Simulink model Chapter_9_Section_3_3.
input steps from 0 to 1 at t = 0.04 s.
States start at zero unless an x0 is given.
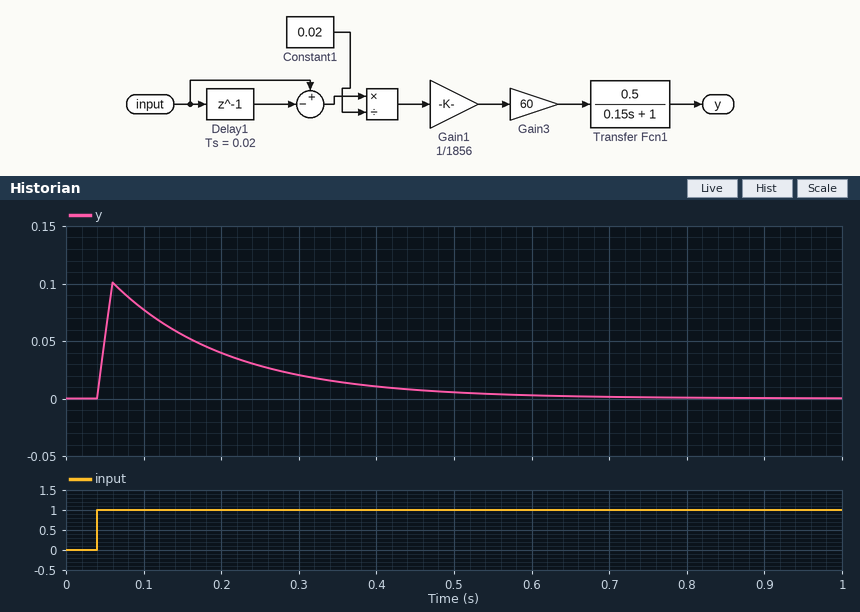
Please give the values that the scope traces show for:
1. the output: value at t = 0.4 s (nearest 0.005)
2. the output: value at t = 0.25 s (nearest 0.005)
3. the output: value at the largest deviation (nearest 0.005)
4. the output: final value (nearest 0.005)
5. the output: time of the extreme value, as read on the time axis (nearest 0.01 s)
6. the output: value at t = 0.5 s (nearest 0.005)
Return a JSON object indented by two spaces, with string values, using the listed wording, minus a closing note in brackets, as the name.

{
  "the output: value at t = 0.4 s": "0.010",
  "the output: value at t = 0.25 s": "0.030",
  "the output: value at the largest deviation": "0.100",
  "the output: final value": "0.000",
  "the output: time of the extreme value, as read on the time axis": "0.06 s",
  "the output: value at t = 0.5 s": "0.005"
}
